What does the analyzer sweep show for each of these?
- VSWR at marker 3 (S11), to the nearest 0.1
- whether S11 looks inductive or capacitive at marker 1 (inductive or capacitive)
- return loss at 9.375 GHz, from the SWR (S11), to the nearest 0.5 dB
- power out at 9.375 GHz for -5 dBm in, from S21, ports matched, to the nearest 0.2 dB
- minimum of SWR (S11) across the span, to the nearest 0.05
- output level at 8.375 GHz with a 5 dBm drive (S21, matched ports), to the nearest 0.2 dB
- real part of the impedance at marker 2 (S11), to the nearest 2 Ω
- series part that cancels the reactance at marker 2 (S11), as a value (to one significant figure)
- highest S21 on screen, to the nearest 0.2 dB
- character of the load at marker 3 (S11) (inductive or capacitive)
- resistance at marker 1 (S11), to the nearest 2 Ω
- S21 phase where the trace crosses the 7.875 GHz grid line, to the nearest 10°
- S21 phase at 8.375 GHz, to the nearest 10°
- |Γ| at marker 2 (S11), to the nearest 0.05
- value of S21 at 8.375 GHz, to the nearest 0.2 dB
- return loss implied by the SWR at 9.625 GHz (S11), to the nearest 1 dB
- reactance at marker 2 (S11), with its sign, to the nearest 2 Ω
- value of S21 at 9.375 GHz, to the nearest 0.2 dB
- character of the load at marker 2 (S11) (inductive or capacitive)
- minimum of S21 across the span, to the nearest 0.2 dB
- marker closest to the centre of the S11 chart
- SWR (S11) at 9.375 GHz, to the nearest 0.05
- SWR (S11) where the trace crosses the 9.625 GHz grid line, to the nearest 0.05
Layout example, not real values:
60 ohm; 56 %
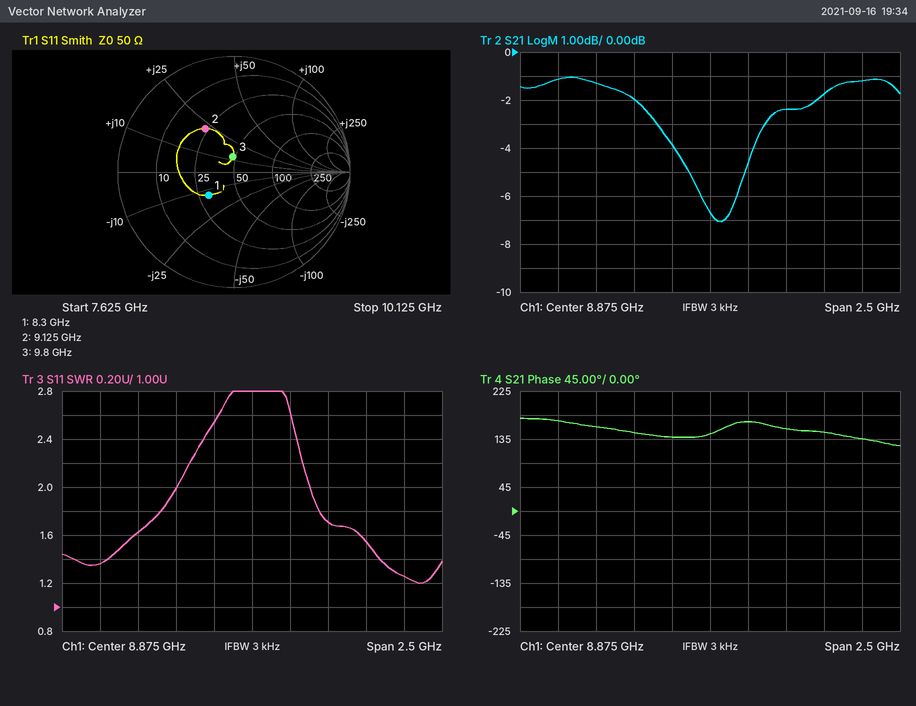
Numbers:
1.3; capacitive; 11.5 dB; -7.4 dBm; 1.20; 3.0 dBm; 24 Ω; 800 fF; -1.0 dB; inductive; 30 Ω; 170°; 150°; 0.45; -2.0 dB; 13 dB; +22 Ω; -2.4 dB; inductive; -7.0 dB; marker 3; 1.70; 1.55
